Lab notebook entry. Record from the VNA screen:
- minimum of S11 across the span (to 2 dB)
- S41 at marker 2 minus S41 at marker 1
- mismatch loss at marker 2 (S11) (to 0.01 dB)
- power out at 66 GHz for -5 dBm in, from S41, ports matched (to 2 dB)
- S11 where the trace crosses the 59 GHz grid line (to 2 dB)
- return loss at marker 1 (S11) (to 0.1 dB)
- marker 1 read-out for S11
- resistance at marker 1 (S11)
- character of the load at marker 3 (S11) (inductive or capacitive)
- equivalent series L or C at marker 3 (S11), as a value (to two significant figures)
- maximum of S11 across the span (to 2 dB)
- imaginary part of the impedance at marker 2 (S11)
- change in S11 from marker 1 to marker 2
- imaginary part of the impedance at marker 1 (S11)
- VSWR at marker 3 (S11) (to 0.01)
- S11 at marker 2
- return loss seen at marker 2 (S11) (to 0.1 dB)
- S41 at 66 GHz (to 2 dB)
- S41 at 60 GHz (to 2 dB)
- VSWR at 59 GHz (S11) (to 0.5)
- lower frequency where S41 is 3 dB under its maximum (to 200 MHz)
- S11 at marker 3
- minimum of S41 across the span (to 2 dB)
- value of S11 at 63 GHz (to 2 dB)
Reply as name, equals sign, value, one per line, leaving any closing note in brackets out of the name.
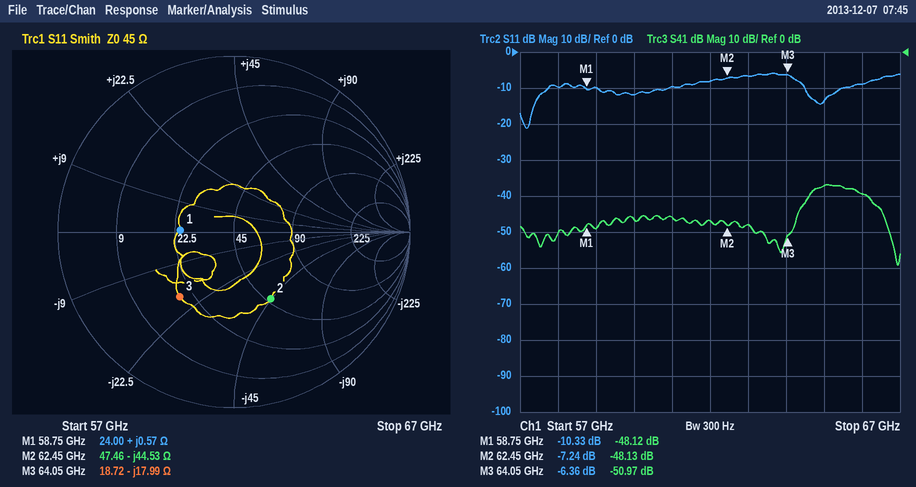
minimum of S11 across the span = -22 dB
S41 at marker 2 minus S41 at marker 1 = -0.01 dB
mismatch loss at marker 2 (S11) = 0.91 dB
power out at 66 GHz for -5 dBm in, from S41, ports matched = -44 dBm
S11 where the trace crosses the 59 GHz grid line = -10 dB
return loss at marker 1 (S11) = 10.3 dB
marker 1 read-out for S11 = -10.33 dB
resistance at marker 1 = 24.00 Ω
character of the load at marker 3 (S11) = capacitive
equivalent series L or C at marker 3 (S11), as a value = 140 fF
maximum of S11 across the span = -6 dB
imaginary part of the impedance at marker 2 = -44.53 Ω
change in S11 from marker 1 to marker 2 = 3.09 dB
imaginary part of the impedance at marker 1 = +0.57 Ω
VSWR at marker 3 (S11) = 2.85
S11 at marker 2 = -7.24 dB
return loss seen at marker 2 (S11) = 7.2 dB
S41 at 66 GHz = -40 dB
S41 at 60 GHz = -46 dB
VSWR at 59 GHz (S11) = 2.0
lower frequency where S41 is 3 dB under its maximum = 64.6 GHz
S11 at marker 3 = -6.36 dB
minimum of S41 across the span = -60 dB
value of S11 at 63 GHz = -6 dB
